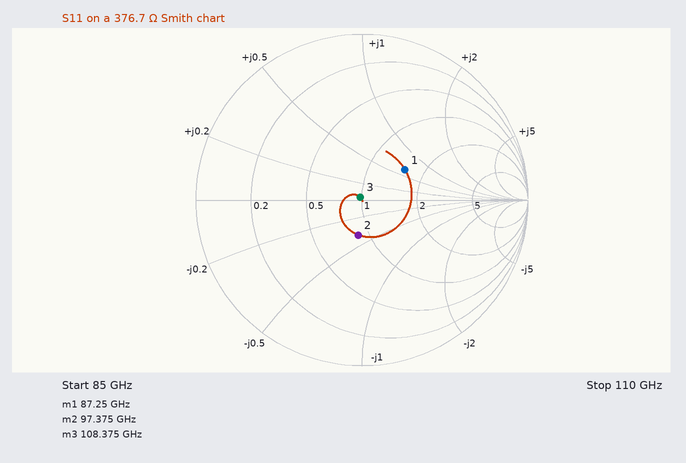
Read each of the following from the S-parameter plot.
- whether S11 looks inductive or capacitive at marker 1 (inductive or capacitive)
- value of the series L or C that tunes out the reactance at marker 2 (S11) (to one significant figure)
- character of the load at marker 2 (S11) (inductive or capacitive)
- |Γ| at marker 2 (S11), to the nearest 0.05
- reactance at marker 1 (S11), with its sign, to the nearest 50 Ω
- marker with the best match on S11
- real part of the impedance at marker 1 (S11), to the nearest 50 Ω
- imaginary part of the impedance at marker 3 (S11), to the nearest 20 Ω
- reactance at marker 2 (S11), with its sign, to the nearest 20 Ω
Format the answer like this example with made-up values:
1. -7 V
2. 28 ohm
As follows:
1. inductive
2. 200 pH
3. capacitive
4. 0.20
5. +250 Ω
6. marker 3
7. 600 Ω
8. +20 Ω
9. -140 Ω
